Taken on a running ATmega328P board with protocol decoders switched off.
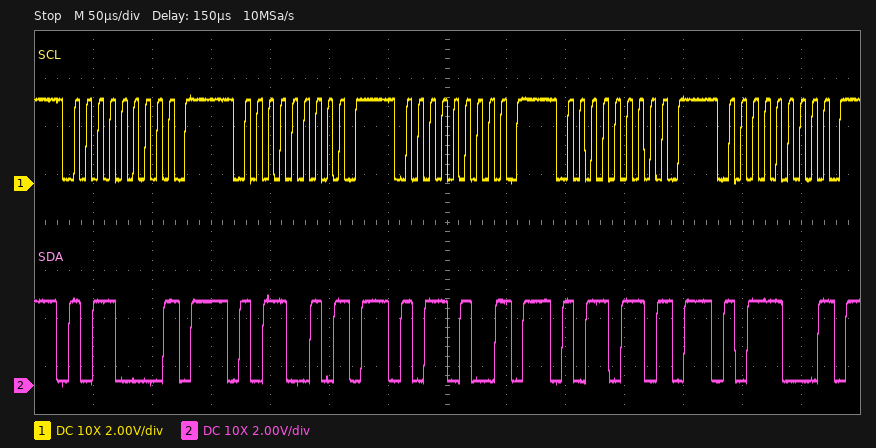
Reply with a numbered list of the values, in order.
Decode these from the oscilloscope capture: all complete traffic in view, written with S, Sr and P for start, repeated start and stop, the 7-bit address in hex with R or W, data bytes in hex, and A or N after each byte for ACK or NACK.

1. S 58W N P S 59W N P S 5AW N P S 5BW N P S 5CW N P
